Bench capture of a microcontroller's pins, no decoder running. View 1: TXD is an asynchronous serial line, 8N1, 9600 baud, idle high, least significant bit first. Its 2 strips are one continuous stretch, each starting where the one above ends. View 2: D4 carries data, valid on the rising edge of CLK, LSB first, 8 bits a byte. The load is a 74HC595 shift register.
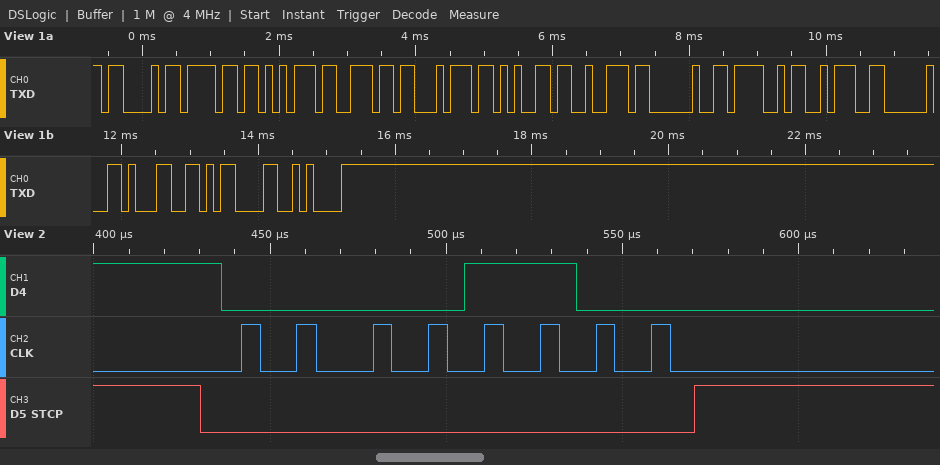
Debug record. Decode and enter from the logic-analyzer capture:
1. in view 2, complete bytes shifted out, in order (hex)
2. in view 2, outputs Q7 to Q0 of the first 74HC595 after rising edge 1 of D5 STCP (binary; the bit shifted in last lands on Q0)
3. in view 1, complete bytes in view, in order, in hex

30
00001100
43 6F 75 6E 74 65 72 20 4F 3A 20 31 0D 0A
